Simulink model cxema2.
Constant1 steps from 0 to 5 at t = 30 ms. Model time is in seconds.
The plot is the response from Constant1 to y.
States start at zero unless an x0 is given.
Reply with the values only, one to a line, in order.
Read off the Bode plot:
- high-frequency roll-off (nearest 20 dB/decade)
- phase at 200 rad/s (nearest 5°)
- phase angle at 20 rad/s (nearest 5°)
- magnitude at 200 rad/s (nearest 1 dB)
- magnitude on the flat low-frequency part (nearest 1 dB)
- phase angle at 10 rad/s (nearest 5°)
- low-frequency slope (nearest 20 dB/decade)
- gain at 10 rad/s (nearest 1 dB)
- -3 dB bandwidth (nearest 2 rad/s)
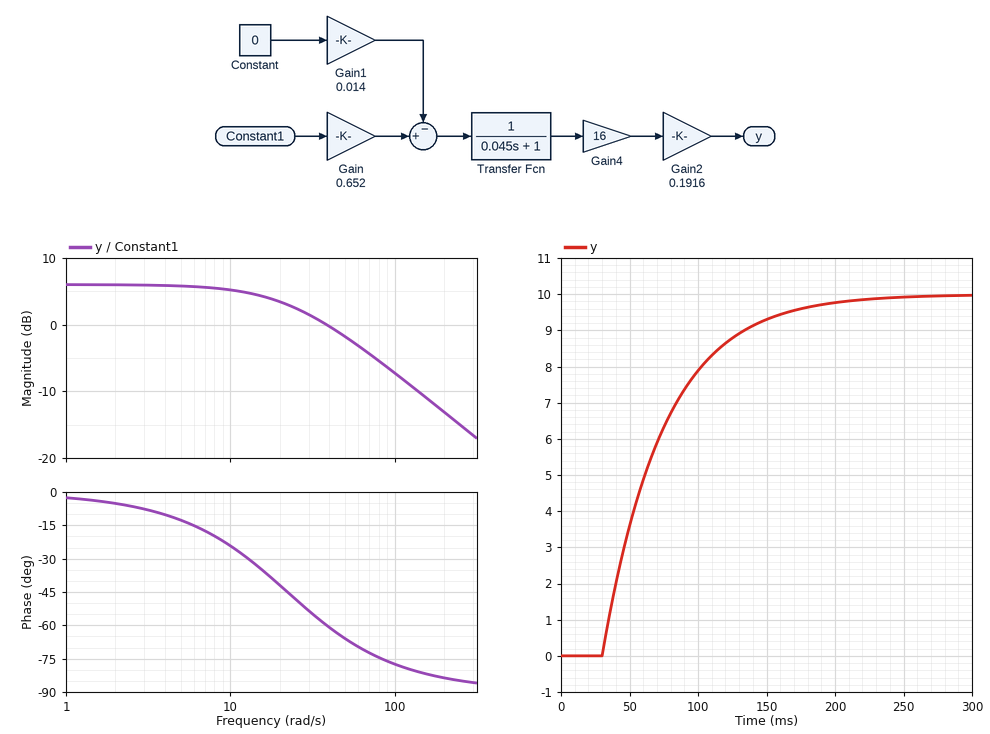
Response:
-20 dB/decade
-85°
-40°
-13 dB
6 dB
-25°
0 dB/decade
5 dB
22 rad/s
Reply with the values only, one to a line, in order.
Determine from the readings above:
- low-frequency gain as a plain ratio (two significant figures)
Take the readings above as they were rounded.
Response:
2.0
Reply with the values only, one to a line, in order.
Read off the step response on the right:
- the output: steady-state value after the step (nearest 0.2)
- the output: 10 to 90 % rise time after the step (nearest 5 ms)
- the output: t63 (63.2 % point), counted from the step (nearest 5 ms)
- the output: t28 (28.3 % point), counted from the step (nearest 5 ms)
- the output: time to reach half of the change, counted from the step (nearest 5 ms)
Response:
10.0
100 ms
45 ms
15 ms
30 ms
